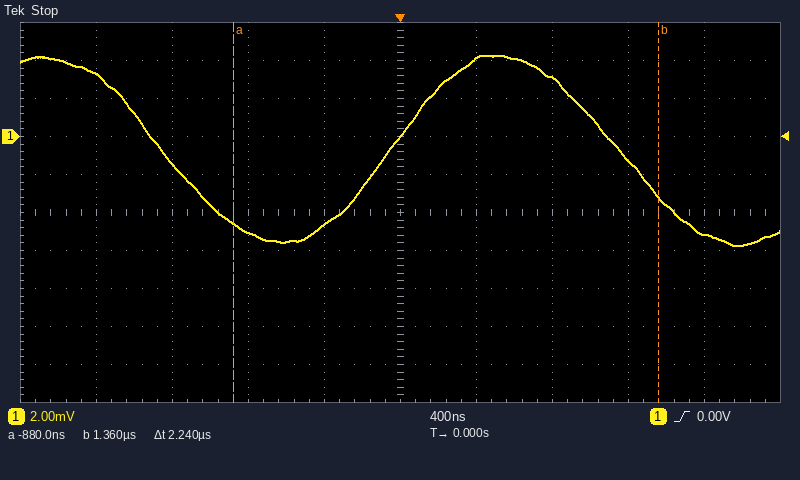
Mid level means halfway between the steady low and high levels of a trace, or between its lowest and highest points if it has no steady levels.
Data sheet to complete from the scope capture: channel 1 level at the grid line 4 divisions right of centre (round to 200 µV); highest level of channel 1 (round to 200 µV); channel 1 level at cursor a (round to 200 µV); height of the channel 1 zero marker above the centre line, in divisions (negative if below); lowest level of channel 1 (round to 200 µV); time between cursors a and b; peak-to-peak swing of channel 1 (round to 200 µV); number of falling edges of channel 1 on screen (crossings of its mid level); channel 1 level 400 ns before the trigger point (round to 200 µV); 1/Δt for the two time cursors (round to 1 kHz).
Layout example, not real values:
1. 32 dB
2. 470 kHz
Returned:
1. -5.2 mV
2. 4.2 mV
3. -4.6 mV
4. +2.0 div
5. -5.8 mV
6. 2.24 µs
7. 10.0 mV
8. 2
9. -4.6 mV
10. 446 kHz
